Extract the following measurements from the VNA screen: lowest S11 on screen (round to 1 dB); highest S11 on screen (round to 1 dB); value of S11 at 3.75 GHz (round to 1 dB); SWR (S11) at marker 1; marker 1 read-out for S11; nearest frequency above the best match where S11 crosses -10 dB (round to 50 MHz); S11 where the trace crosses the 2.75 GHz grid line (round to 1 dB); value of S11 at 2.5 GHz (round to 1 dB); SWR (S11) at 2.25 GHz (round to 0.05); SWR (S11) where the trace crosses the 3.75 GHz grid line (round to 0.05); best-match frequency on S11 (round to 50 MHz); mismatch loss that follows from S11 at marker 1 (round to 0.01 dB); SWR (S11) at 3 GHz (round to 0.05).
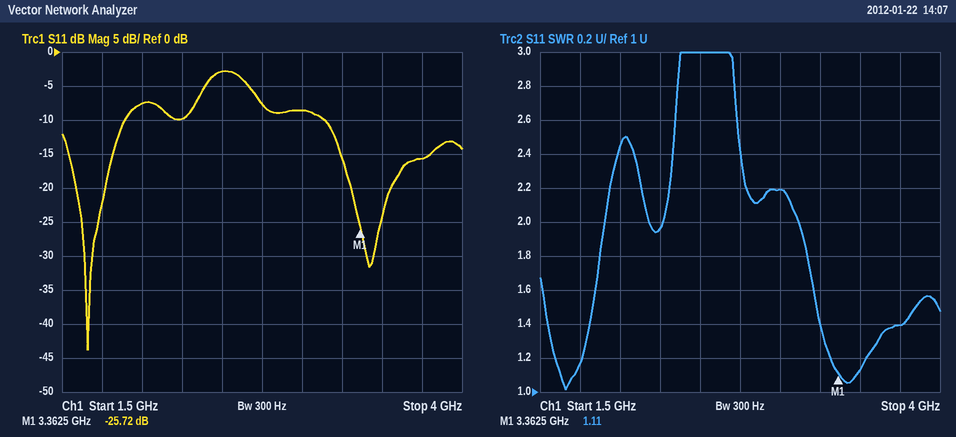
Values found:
-44 dB
-3 dB
-16 dB
1.11
-25.72 dB
1.90 GHz
-8 dB
-3 dB
1.95
1.40
1.65 GHz
0.01 dB
2.20
